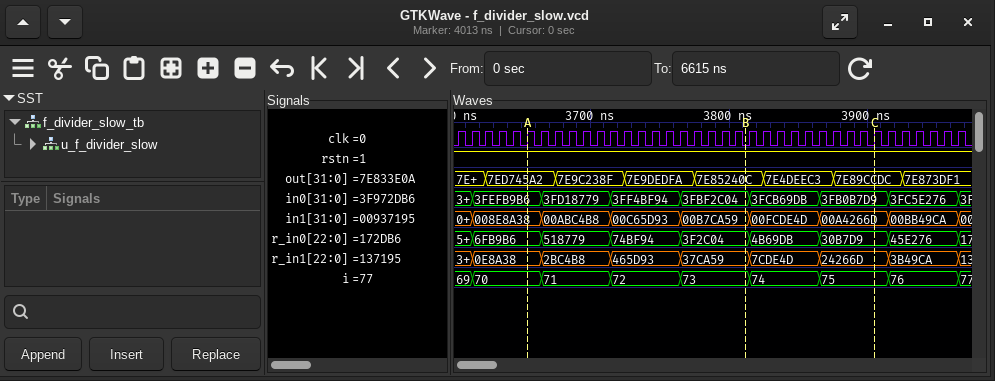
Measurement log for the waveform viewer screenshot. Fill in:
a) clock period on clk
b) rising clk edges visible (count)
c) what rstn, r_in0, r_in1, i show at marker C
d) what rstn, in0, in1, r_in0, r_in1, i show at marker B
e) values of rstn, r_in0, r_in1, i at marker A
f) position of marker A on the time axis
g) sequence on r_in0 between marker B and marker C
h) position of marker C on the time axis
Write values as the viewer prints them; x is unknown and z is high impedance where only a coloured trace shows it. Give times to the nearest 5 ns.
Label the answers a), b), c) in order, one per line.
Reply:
a) 10 ns
b) 37
c) rstn=1, r_in0=30B7D9, r_in1=24266D, i=75
d) rstn=1, in0=3FBF2C04, in1=00B7CA59, r_in0=3F2C04, r_in1=37CA59, i=73
e) rstn=1, r_in0=6FB9B6, r_in1=0E8A38, i=70
f) 3655 ns
g) 3F2C04, 4B69DB, 30B7D9
h) 3905 ns
